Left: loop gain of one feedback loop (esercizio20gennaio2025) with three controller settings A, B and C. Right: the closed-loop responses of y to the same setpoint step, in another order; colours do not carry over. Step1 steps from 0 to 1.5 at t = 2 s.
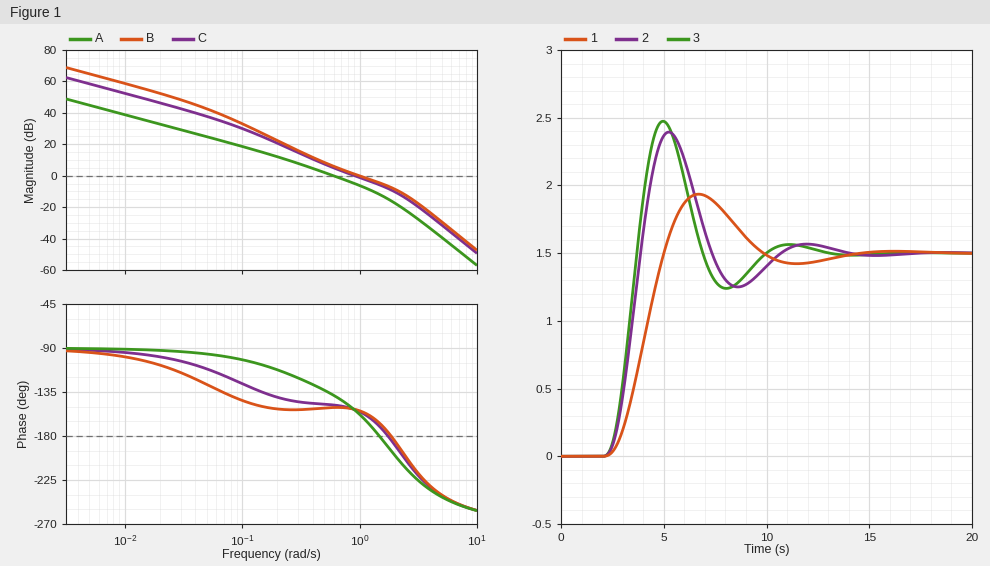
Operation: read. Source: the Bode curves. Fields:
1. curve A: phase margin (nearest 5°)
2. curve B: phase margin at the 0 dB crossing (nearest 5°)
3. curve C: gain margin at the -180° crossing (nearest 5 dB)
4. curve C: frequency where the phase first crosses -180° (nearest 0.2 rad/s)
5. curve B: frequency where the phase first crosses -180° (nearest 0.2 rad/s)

40°
25°
10 dB
1.8 rad/s
1.8 rad/s
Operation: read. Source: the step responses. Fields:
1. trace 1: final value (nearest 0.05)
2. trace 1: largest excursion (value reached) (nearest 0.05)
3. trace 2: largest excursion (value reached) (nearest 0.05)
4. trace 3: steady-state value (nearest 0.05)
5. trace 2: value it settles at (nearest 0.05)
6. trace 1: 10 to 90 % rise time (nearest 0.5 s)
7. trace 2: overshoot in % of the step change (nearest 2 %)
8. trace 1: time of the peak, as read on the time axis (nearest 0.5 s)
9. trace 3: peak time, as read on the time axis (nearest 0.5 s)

1.50
1.95
2.40
1.50
1.50
2.0 s
60 %
6.5 s
5.0 s
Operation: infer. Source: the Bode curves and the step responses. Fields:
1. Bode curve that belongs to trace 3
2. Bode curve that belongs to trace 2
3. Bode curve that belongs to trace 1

B
C
A
